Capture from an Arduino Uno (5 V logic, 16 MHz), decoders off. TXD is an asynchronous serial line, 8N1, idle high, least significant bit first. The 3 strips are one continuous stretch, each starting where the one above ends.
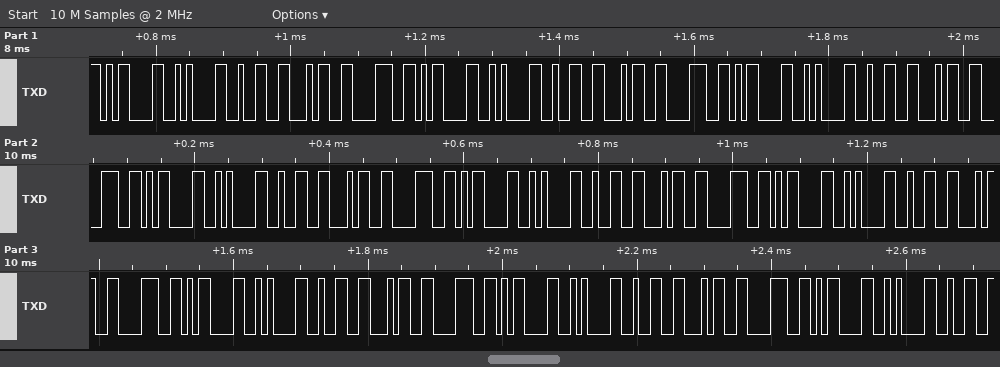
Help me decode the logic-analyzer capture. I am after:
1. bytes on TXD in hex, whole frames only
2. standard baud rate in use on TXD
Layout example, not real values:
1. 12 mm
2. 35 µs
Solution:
1. 0x0D 0x0A 0x32 0x34 0x38 0x0D 0x0A 0x32 0x34 0x38 0x0D 0x0A 0x32 0x34 0x38 0x0D 0x0A 0x32 0x34 0x38 0x0D 0x0A 0x32 0x34 0x38 0x0D 0x0A 0x32 0x34 0x38 0x0D 0x0A 0x32 0x34 0x38 0x0D 0x0A 0x32 0x34 0x38 0x0D 0x0A 0x32
2. 115200 baud
